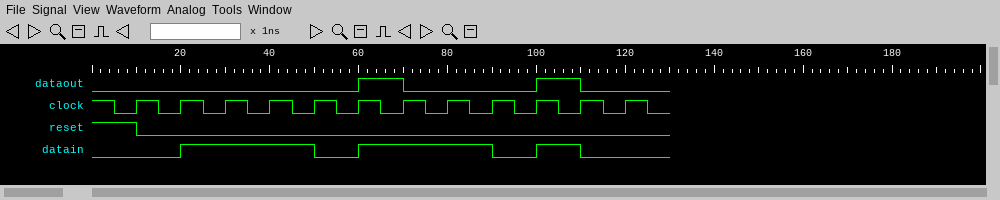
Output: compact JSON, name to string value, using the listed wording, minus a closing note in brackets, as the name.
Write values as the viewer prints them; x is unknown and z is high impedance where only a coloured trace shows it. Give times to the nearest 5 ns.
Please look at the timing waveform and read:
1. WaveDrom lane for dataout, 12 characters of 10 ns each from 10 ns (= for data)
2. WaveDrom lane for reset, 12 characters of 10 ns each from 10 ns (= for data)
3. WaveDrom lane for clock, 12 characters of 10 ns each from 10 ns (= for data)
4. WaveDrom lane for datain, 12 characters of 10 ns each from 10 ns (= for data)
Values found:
{"WaveDrom lane for dataout, 12 characters of 10 ns each from 10 ns": "{name: 'dataout', wave: '0....10..10.'}", "WaveDrom lane for reset, 12 characters of 10 ns each from 10 ns": "{name: 'reset', wave: '0...........'}", "WaveDrom lane for clock, 12 characters of 10 ns each from 10 ns": "{name: 'clock', wave: 'p...........'}", "WaveDrom lane for datain, 12 characters of 10 ns each from 10 ns": "{name: 'datain', wave: '01..01..010.'}"}
